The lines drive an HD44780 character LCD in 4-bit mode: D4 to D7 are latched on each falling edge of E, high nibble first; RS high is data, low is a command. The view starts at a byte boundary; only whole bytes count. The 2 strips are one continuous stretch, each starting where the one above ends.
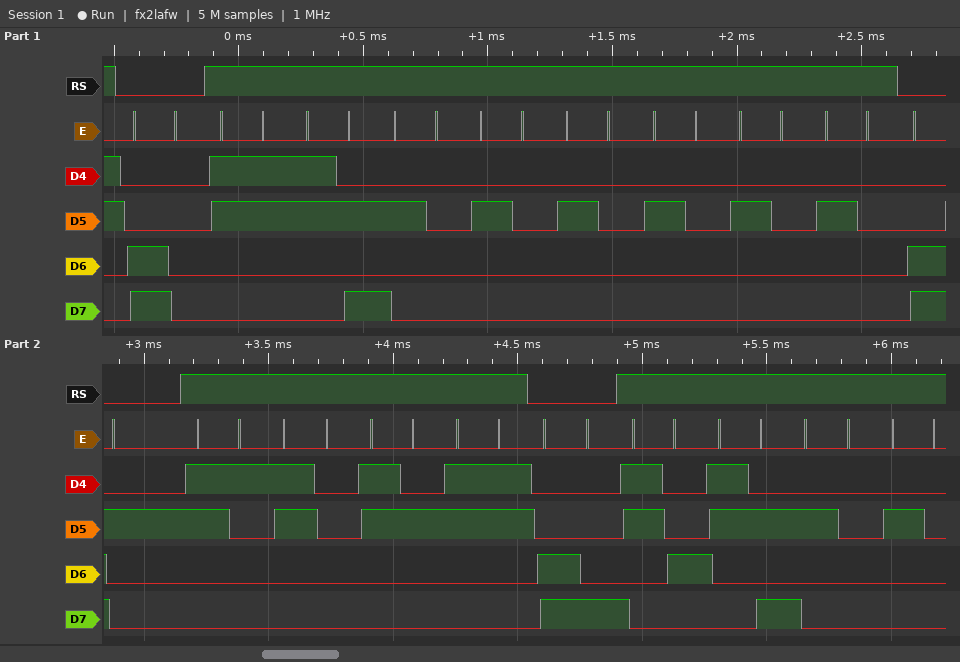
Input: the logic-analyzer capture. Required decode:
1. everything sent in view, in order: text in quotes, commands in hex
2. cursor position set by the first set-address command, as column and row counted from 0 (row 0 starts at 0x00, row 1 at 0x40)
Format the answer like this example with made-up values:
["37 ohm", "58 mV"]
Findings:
["0xC0 \"3:      \" 0xC2 \"1023\" 0xC8 \"4:  \"", "column 0, row 1"]
